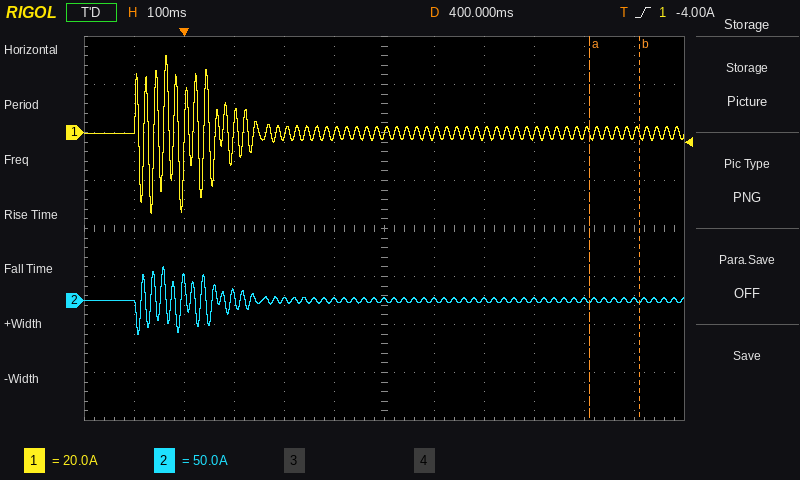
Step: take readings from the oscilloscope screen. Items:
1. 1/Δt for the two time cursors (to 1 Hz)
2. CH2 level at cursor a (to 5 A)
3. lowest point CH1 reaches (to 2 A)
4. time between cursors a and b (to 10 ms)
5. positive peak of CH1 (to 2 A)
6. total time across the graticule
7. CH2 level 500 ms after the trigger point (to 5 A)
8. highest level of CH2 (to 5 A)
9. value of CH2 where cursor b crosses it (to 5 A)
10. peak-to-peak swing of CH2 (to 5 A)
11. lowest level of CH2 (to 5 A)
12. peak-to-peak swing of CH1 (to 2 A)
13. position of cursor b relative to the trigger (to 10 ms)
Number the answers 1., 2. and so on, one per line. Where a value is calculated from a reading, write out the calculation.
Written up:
1. 1 / 100 ms ≈ 10 Hz
2. 0 A
3. -34 A
4. 100 ms
5. 32 A
6. 1.2 s
7. 0 A
8. 35 A
9. 0 A
10. 35 A − (-35 A) = 70 A
11. -35 A
12. 32 A − (-34 A) = 66 A
13. +910 ms
